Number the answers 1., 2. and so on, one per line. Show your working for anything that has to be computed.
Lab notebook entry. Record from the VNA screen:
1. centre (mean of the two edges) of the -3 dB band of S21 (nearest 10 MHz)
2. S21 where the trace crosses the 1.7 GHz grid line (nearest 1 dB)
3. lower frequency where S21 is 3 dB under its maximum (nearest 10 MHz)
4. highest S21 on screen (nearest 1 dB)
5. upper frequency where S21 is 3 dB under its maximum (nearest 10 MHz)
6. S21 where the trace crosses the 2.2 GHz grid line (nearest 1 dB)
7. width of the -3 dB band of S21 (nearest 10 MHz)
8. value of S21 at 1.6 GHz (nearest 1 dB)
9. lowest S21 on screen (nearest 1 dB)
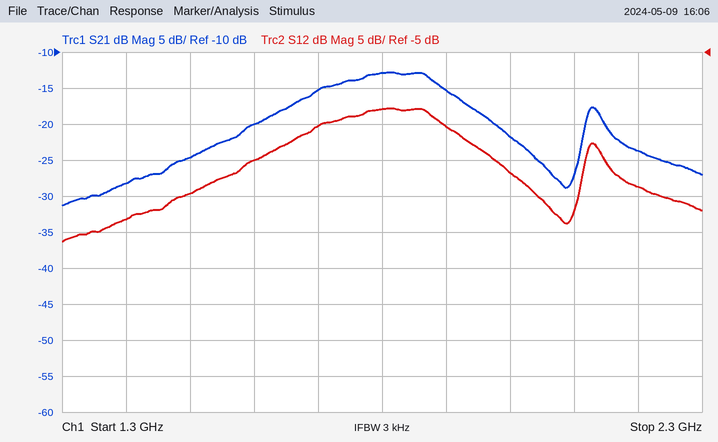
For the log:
1. 1.80 GHz
2. -15 dB
3. 1.69 GHz
4. -13 dB
5. 1.91 GHz
6. -24 dB
7. 1.91 GHz − 1.69 GHz = 220 MHz
8. -20 dB
9. -31 dB
